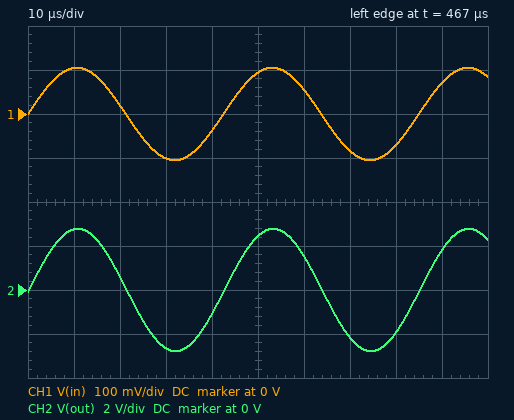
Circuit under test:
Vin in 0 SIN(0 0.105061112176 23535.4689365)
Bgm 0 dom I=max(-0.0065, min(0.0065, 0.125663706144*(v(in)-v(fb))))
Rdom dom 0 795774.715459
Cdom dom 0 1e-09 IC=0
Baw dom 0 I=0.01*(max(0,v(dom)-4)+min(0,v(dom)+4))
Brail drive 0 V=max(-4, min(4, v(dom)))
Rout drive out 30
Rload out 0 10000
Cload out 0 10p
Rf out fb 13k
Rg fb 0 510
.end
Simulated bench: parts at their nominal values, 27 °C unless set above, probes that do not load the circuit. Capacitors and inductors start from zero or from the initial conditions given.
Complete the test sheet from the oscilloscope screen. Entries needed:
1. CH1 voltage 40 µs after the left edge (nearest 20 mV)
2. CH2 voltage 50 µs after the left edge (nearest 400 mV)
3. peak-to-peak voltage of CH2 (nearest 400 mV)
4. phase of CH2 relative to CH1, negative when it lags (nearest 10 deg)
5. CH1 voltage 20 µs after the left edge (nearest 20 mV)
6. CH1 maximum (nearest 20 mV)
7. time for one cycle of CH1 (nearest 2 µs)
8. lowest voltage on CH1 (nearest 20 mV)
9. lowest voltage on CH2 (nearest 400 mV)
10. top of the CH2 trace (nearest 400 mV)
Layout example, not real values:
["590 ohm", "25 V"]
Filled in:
["-40 mV", "2.4 V", "5.6 V", "0 deg", "20 mV", "100 mV", "42 µs", "-100 mV", "-2.8 V", "2.8 V"]
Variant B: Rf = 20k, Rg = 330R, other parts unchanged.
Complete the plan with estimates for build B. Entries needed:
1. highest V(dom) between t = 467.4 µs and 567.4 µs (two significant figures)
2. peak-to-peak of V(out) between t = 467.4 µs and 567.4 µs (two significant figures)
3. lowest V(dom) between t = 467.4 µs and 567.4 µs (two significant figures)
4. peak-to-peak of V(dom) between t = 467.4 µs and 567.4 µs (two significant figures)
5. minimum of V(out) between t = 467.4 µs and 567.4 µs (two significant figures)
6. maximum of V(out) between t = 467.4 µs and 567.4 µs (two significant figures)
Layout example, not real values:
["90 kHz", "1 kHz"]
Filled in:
["4.5 V", "8.0 V", "-4.5 V", "9.0 V", "-4.0 V", "4.0 V"]
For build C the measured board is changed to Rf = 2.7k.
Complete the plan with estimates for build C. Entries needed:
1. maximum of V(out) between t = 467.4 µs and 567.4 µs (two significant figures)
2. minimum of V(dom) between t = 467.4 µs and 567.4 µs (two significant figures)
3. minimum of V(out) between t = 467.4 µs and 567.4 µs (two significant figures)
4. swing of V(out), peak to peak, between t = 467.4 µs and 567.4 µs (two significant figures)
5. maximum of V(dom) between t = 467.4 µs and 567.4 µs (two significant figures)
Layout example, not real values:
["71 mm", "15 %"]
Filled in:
["660 mV", "-670 mV", "-660 mV", "1.3 V", "670 mV"]
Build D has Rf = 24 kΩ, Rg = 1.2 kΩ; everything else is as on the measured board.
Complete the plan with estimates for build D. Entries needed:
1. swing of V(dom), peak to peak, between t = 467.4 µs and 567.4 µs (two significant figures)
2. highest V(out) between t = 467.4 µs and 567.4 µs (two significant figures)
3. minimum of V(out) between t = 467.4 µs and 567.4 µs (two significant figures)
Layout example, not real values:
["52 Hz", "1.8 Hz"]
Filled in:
["4.4 V", "2.2 V", "-2.2 V"]
